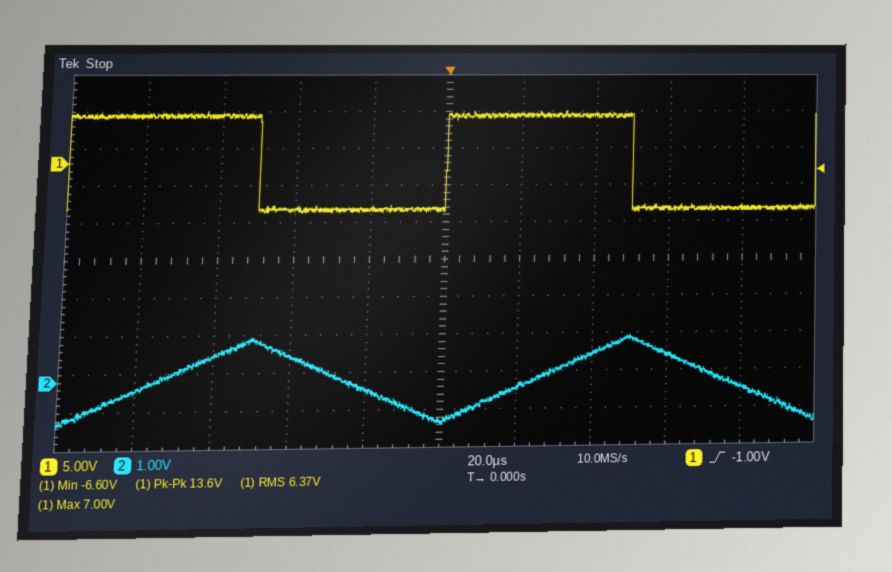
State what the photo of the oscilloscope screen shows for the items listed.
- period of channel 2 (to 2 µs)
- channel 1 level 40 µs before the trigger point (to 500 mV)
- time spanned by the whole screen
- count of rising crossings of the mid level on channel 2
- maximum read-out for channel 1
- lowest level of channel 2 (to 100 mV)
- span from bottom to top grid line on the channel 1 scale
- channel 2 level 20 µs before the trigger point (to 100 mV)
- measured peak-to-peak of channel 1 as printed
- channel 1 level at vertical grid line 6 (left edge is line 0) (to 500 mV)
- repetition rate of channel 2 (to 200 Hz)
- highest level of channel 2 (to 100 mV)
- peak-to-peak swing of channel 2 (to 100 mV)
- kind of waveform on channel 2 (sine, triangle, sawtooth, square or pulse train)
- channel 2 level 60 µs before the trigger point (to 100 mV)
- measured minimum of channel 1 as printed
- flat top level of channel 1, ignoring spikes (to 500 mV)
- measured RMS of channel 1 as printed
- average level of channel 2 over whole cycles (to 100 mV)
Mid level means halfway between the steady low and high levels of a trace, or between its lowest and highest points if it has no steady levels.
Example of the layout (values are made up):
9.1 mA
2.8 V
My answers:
100 µs
-6.0 V
200 µs
2
7.00 V
-1.2 V
50 V
-300 mV
13.6 V
6.5 V
10.0 kHz
1.1 V
2.3 V
triangle
600 mV
-6.60 V
6.5 V
6.37 V
0.0 V
